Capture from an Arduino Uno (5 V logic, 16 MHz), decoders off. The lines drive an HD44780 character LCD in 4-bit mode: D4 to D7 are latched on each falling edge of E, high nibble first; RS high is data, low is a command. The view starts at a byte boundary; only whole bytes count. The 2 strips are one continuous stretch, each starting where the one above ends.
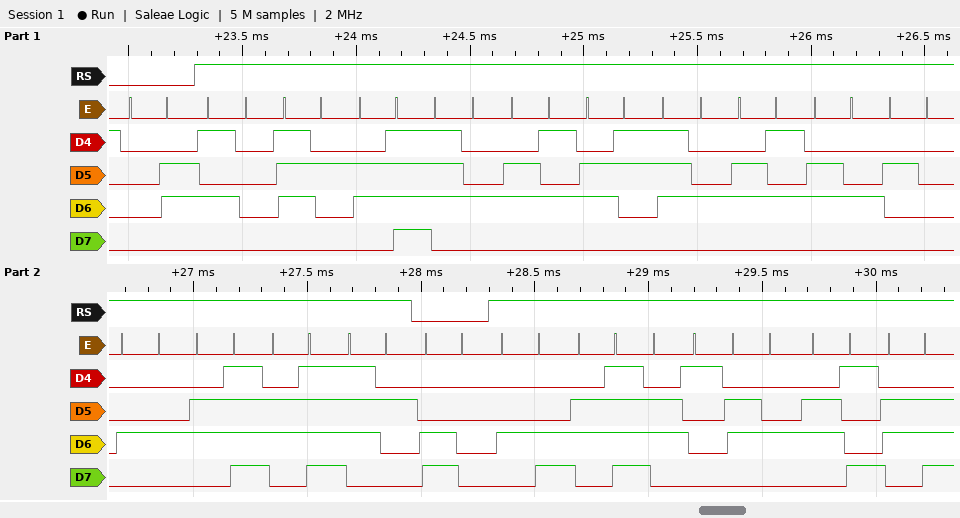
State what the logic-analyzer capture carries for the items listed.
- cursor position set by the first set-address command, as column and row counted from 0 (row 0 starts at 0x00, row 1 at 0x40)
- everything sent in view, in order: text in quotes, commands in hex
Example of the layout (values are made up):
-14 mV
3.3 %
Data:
column 0, row 1
0x06 "Protected Door" 0xC0 "Loadin"
